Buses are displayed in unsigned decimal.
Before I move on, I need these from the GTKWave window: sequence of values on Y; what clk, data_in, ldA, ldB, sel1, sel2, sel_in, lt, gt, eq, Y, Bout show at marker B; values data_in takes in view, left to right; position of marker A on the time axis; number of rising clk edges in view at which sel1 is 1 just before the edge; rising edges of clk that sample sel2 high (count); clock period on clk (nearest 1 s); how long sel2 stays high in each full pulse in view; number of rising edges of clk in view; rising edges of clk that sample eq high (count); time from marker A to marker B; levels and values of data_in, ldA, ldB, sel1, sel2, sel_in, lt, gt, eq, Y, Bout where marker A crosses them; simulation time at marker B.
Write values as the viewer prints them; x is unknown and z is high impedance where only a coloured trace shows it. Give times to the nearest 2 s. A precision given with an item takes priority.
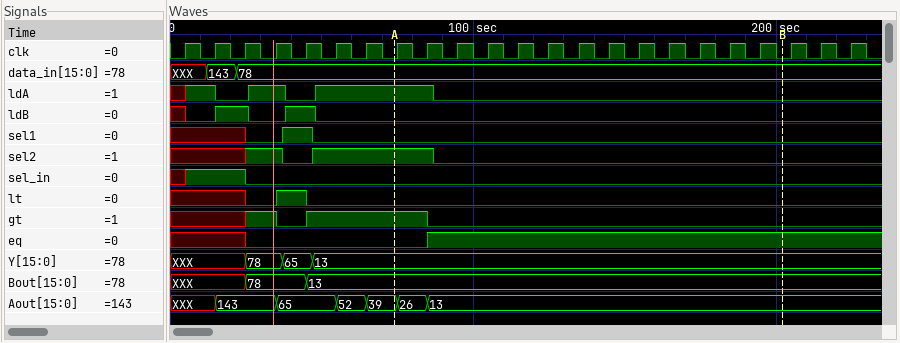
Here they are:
XXX, 78, 65, 13
clk=0, data_in=78, ldA=0, ldB=0, sel1=0, sel2=0, sel_in=0, lt=0, gt=0, eq=1, Y=13, Bout=13
XXX, 143, 78
74 s
1
5
10 s
40 s
23
14
128 s
data_in=78, ldA=1, ldB=0, sel1=0, sel2=1, sel_in=0, lt=0, gt=1, eq=0, Y=13, Bout=13
202 s
